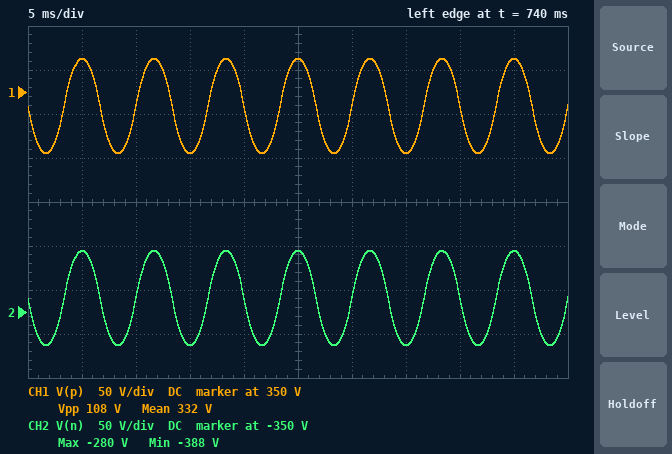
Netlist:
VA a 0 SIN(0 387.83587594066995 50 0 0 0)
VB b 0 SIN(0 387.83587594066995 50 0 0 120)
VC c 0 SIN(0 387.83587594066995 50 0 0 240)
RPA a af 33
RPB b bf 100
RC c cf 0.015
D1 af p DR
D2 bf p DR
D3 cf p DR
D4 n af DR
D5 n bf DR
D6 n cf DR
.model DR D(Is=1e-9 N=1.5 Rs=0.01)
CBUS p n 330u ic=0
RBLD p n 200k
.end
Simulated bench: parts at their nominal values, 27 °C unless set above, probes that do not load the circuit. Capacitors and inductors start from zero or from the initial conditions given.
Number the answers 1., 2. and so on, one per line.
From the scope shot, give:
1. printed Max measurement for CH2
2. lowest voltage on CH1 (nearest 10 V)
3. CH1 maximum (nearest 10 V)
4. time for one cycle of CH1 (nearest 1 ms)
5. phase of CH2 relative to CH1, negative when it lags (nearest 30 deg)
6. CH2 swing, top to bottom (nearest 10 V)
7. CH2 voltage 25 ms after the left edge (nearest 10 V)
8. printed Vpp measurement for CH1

1. -280 V
2. 280 V
3. 390 V
4. 7 ms
5. 0 deg
6. 110 V
7. -280 V
8. 108 V
